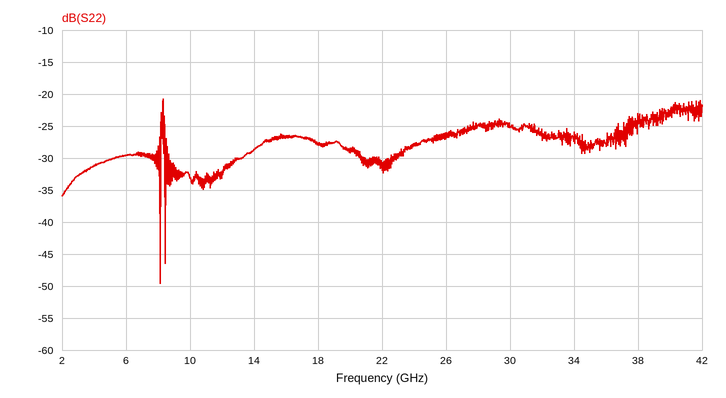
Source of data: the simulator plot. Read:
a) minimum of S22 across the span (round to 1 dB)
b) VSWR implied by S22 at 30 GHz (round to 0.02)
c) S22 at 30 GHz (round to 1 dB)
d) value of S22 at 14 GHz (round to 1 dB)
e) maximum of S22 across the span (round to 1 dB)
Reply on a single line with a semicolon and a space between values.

-50 dB; 1.12; -25 dB; -29 dB; -21 dB
